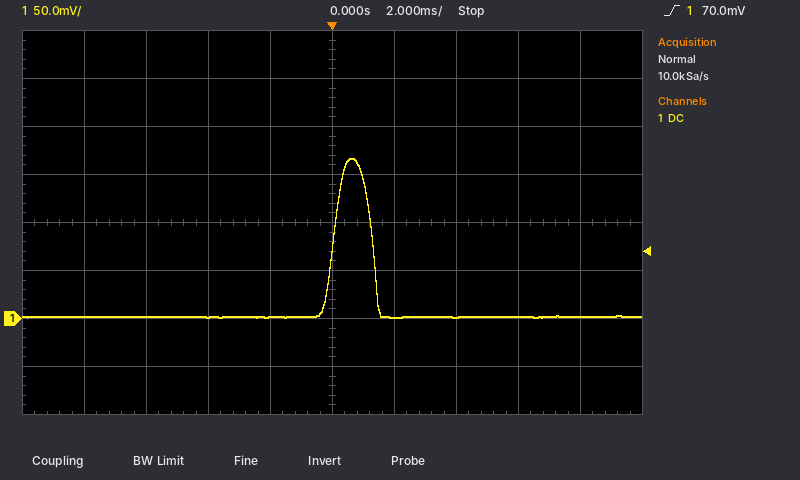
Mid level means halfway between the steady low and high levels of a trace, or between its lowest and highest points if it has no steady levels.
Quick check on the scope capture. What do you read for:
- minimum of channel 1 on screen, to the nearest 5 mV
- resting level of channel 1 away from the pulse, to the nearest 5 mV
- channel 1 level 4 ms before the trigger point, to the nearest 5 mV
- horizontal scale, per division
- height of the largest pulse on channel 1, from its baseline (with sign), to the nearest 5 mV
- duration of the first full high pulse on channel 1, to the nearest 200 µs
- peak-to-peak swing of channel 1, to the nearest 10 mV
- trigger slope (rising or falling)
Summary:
0 mV
0 mV
0 mV
2 ms
+165 mV
1.2 ms
170 mV
rising
